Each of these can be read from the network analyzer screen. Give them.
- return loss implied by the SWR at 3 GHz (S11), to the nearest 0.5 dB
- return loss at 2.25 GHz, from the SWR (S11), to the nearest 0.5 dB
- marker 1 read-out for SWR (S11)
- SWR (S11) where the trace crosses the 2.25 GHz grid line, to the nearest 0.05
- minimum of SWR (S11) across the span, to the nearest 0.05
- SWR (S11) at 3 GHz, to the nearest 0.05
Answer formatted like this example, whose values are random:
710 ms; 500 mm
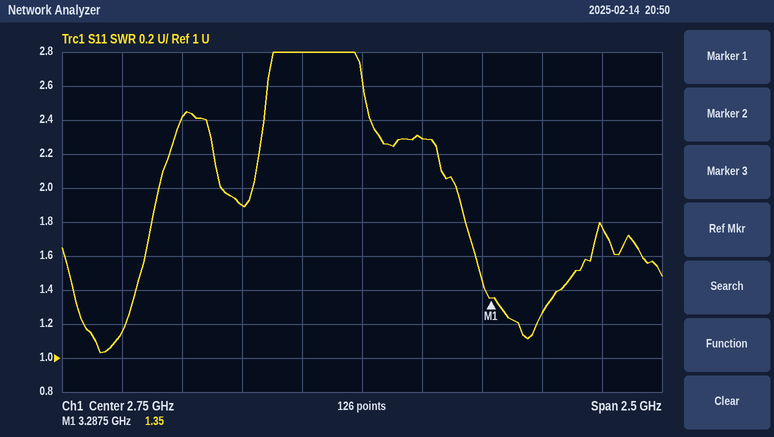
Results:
8.0 dB; 10.0 dB; 1.35; 1.90; 1.05; 2.30
